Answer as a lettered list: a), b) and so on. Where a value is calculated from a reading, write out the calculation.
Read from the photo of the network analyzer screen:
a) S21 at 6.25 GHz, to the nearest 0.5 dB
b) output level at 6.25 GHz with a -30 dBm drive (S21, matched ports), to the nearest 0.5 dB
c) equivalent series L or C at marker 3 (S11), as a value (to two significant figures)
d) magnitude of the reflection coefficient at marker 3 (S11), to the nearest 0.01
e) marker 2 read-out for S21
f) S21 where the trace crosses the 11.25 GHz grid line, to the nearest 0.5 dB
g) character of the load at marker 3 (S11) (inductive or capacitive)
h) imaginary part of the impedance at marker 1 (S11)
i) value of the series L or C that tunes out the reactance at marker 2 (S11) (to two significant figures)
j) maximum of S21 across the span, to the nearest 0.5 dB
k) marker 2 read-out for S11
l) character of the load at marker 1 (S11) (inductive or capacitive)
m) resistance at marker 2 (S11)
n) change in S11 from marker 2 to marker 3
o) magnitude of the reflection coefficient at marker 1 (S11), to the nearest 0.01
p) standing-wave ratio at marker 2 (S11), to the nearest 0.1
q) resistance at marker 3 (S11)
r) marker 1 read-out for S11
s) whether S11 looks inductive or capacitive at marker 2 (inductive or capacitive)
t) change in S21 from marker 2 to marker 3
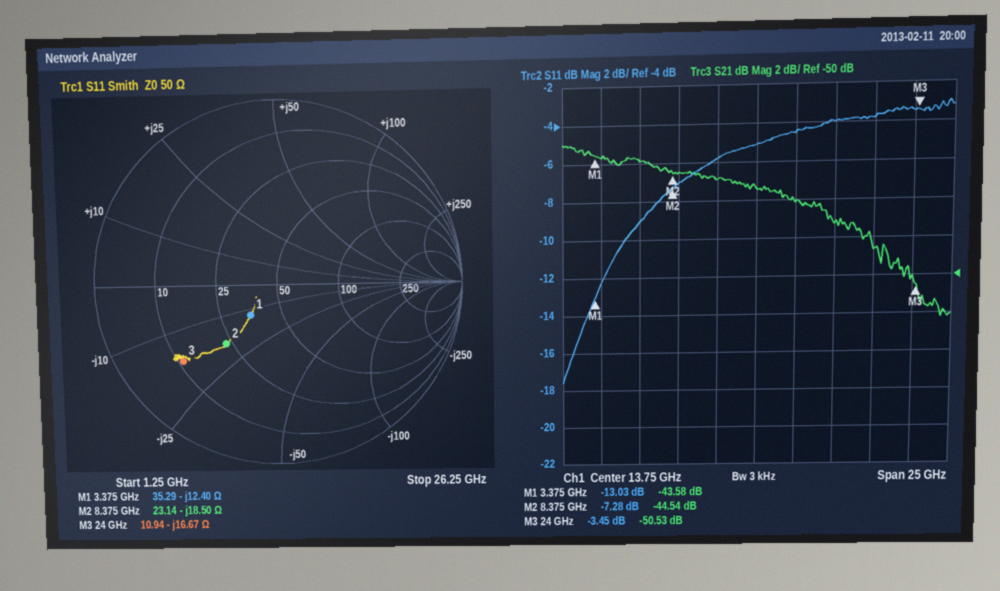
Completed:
a) -44.0 dB
b) -30 dBm + (-44.0 dB) = -74.0 dBm
c) C = 1/(2π × 24 GHz × 16.67 Ω) ≈ 398 fF, so 400 fF to two significant figures
d) 0.67
e) -44.54 dB
f) -45.0 dB
g) capacitive
h) -12.40 Ω
i) L = 18.5 Ω/(2π × 8.375 GHz) ≈ 352 pH, so 350 pH to two significant figures
j) -43.0 dB
k) -7.28 dB
l) capacitive
m) 23.14 Ω
n) -3.45 − (-7.28) = 3.83 dB
o) 10^(-13.03/20) ≈ 0.22
p) 2.5
q) 10.94 Ω
r) -13.03 dB
s) capacitive
t) -50.53 − (-44.54) = -5.99 dB
